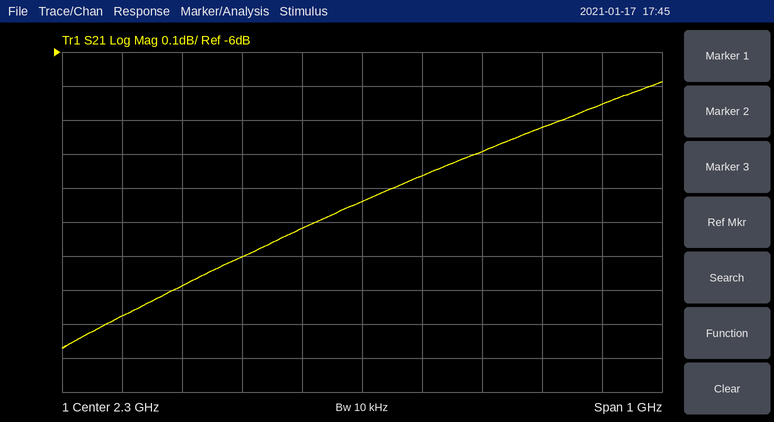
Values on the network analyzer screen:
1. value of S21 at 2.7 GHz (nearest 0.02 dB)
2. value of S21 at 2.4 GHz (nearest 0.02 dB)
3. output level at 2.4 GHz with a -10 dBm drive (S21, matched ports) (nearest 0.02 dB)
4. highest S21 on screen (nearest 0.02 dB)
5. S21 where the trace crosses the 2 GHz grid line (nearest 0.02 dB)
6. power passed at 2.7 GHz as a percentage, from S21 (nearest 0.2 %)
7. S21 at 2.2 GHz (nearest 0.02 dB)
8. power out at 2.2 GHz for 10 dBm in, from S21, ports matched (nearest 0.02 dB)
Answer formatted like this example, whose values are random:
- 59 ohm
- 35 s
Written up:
- -6.16 dB
- -6.36 dB
- -16.36 dBm
- -6.08 dB
- -6.68 dB
- 24.2 %
- -6.52 dB
- 3.48 dBm
